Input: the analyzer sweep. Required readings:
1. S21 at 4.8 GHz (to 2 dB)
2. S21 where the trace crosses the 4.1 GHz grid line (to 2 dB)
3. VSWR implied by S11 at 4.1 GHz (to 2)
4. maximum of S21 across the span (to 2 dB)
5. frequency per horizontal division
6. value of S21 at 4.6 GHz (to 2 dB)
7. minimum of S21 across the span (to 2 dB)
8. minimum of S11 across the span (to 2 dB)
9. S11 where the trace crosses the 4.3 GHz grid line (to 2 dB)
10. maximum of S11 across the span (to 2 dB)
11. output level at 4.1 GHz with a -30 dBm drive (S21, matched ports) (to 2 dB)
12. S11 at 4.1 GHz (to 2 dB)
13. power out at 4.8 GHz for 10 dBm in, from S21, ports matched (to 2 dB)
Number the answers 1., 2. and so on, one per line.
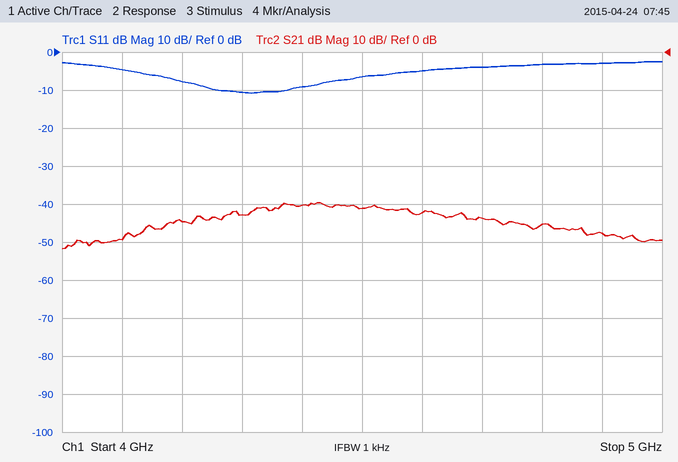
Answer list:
1. -46 dB
2. -50 dB
3. 4
4. -40 dB
5. 100 MHz
6. -42 dB
7. -52 dB
8. -10 dB
9. -10 dB
10. -2 dB
11. -80 dBm
12. -4 dB
13. -36 dBm
